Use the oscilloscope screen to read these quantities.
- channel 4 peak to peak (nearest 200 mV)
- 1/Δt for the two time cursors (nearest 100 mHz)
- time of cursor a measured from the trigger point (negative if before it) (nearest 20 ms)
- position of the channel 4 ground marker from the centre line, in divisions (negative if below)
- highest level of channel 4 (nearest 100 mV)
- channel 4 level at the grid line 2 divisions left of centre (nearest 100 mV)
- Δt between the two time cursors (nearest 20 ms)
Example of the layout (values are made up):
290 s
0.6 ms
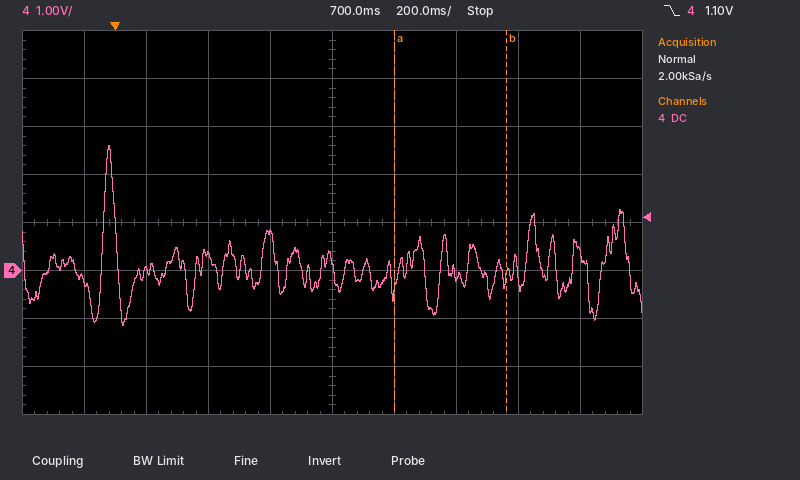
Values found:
3.8 V
2.8 Hz
+900 ms
-1.0 div
2.6 V
300 mV
360 ms
